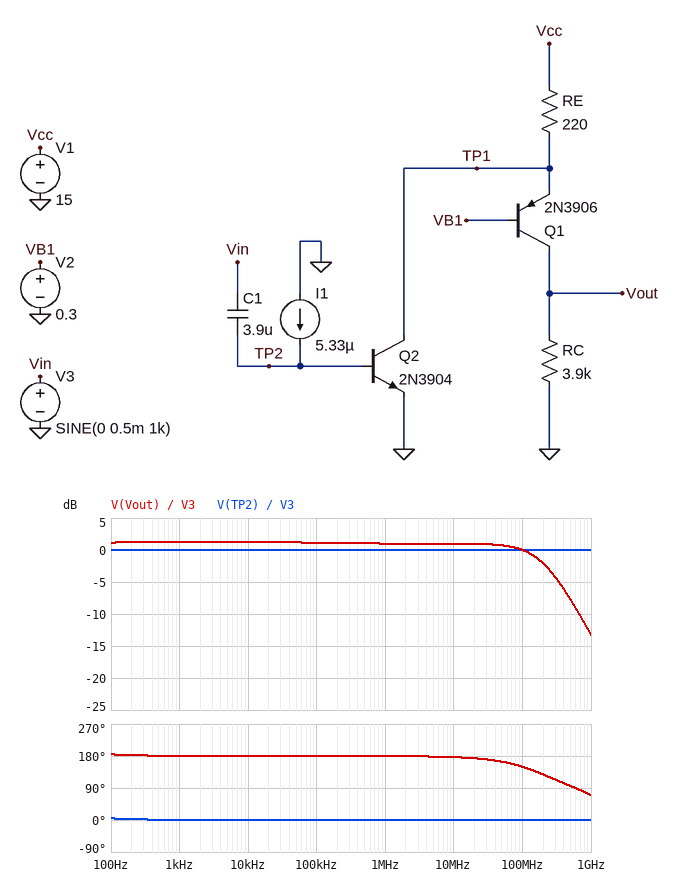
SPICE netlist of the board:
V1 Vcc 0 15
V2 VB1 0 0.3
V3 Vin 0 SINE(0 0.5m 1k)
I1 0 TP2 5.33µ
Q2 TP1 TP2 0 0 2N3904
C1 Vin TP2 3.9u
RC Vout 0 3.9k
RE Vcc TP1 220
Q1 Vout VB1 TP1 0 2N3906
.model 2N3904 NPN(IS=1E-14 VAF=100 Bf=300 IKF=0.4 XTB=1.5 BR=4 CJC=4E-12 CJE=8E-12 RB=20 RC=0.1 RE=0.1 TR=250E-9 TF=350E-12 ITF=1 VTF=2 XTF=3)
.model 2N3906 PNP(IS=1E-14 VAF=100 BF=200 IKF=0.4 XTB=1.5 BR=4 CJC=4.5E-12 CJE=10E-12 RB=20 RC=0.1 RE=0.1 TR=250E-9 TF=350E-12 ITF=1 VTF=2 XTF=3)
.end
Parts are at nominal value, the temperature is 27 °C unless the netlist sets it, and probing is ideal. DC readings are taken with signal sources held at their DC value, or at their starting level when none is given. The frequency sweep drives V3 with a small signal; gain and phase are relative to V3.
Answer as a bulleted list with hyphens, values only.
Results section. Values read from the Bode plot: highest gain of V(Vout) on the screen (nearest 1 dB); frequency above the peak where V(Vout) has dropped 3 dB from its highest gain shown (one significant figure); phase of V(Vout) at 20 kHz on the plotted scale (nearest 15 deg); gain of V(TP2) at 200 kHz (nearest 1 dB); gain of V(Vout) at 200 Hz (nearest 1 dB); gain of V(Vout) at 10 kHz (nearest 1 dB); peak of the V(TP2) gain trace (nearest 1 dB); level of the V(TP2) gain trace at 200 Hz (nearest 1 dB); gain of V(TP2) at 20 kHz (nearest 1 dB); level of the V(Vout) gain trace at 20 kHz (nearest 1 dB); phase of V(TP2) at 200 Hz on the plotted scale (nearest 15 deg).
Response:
- 1 dB
- 200 MHz
- 180 deg
- 0 dB
- 1 dB
- 1 dB
- 0 dB
- 0 dB
- 0 dB
- 1 dB
- 0 deg
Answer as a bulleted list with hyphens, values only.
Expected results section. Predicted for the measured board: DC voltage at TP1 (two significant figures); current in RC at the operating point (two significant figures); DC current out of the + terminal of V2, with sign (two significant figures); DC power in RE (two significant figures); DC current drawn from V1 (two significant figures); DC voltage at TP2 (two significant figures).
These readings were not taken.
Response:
- 2.2 V
- 570 µA
- -56 mA
- 740 mW
- 58 mA
- 670 mV
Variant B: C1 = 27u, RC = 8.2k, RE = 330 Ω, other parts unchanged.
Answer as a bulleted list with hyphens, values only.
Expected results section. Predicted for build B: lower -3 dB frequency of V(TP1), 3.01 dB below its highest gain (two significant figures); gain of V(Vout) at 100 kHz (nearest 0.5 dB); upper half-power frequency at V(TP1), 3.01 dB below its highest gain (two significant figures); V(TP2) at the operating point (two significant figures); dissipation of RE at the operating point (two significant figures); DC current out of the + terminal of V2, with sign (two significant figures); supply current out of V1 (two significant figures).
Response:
- 1.2 Hz
- 1.5 dB
- 180 MHz
- 670 mV
- 520 mW
- -38 mA
- 40 mA
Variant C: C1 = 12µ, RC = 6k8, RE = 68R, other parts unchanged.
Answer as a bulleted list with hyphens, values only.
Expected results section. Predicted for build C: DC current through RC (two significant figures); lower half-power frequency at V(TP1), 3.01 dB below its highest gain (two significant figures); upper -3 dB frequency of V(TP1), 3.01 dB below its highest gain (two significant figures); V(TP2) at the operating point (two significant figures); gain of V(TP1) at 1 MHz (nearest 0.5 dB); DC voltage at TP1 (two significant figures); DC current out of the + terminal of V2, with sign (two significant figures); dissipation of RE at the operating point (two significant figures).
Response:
- 620 µA
- 2.7 Hz
- 200 MHz
- 670 mV
- 0 dB
- 4.3 V
- -160 mA
- 1.7 W
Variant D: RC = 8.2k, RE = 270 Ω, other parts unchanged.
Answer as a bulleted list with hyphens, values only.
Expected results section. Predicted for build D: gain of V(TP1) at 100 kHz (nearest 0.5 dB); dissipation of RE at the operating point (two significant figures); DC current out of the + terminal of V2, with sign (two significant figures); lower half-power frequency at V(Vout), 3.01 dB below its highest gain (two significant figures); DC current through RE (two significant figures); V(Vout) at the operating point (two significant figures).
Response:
- 1.5 dB
- 620 mW
- -46 mA
- 8.3 Hz
- 48 mA
- 2.0 V
